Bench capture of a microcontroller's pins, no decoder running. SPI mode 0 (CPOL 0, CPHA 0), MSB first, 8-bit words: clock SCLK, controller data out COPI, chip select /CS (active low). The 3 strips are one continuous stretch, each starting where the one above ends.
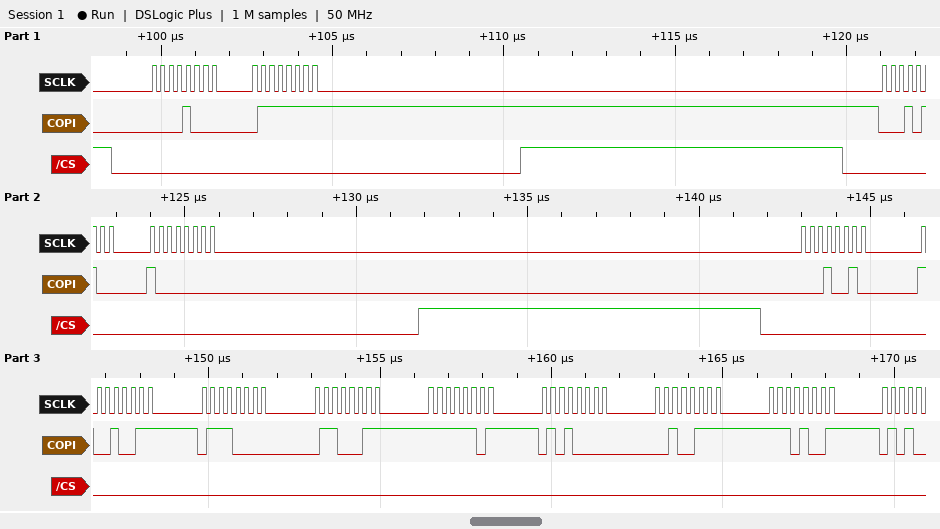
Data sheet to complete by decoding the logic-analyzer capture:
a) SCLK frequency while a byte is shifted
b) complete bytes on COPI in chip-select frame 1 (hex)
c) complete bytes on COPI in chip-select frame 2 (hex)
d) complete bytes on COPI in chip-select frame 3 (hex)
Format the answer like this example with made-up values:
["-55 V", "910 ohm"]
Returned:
["4 MHz", "08 7F", "14 80", "12 93 70 63 FD 50 27 E9"]
